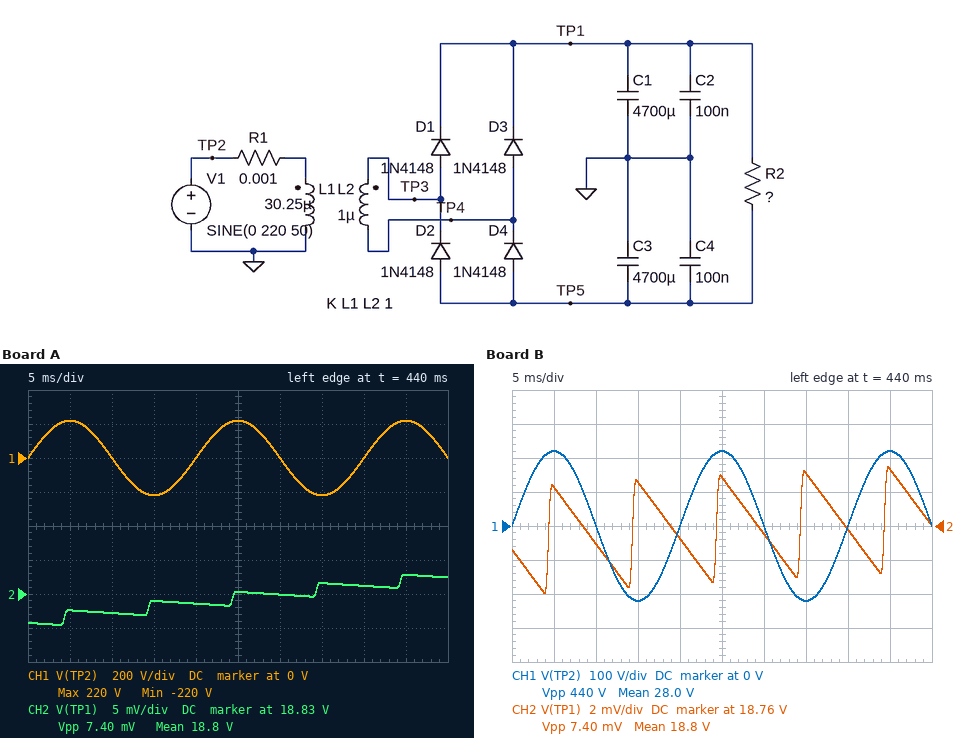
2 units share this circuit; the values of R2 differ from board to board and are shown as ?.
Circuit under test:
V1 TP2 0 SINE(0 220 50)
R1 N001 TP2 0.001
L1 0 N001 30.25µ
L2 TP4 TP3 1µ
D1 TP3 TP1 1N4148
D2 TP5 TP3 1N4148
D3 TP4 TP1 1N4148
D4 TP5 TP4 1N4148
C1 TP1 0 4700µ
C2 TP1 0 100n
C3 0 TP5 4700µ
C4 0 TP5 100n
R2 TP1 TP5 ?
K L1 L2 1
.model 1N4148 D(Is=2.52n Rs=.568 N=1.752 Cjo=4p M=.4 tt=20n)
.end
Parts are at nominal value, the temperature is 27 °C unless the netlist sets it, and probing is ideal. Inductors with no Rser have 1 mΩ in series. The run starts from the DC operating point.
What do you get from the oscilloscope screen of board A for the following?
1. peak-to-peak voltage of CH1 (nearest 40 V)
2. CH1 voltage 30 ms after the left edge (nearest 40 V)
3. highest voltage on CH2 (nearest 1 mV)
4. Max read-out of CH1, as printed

440 V
0 V
18.833 V
220 V
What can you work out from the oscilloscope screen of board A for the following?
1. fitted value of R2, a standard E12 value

100 kΩ
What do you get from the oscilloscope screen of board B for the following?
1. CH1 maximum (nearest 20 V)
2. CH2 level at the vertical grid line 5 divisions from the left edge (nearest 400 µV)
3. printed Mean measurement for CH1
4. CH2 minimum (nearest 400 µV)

220 V
18.7588 V
28.0 V
18.7520 V
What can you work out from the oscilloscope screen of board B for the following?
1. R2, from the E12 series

12 kΩ
